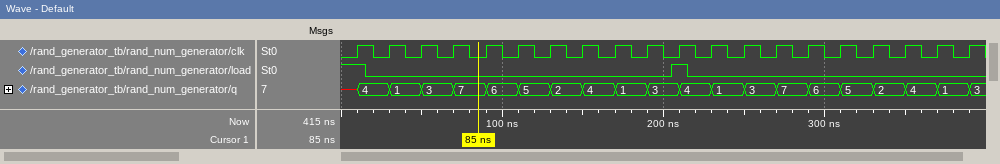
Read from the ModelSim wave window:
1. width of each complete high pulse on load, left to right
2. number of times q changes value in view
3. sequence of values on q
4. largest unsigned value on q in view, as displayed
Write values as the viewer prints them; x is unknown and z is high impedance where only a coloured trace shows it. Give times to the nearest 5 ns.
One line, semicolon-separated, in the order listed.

10 ns; 20; x, 4, 1, 3, 7, 6, 5, 2, 4, 1, 3, 4, 1, 3, 7, 6, 5, 2, 4, 1, 3; 7
